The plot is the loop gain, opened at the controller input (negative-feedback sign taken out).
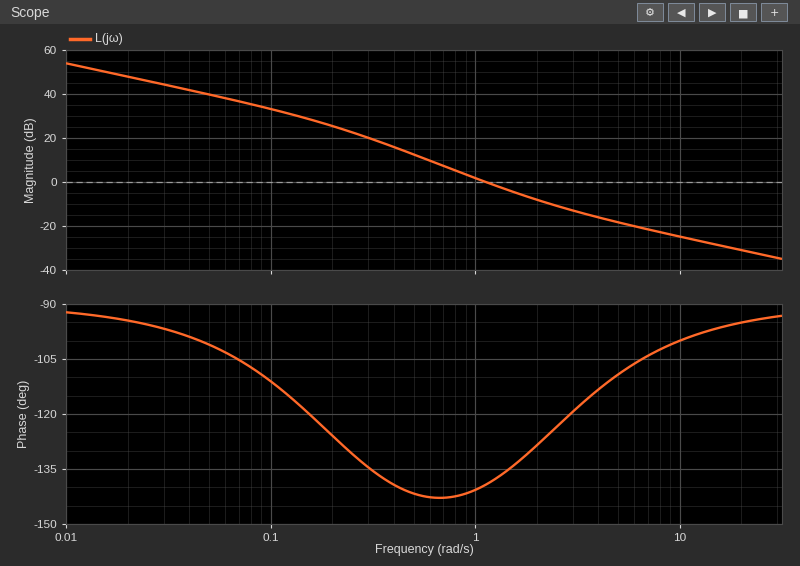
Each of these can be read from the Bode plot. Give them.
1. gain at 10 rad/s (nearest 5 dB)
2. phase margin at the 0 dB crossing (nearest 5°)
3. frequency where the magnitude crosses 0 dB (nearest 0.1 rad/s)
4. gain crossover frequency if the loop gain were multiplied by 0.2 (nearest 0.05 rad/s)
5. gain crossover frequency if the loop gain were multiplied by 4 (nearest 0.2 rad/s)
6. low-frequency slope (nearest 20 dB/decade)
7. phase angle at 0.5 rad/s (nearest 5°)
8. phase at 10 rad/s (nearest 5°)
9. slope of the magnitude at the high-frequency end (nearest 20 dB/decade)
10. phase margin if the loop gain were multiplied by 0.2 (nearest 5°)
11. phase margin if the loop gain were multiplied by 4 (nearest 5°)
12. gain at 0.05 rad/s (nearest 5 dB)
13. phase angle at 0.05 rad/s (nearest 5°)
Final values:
-25 dB
40°
1.1 rad/s
0.45 rad/s
2.8 rad/s
-20 dB/decade
-140°
-100°
-20 dB/decade
40°
60°
40 dB
-100°
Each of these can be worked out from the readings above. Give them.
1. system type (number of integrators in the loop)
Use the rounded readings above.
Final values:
1
